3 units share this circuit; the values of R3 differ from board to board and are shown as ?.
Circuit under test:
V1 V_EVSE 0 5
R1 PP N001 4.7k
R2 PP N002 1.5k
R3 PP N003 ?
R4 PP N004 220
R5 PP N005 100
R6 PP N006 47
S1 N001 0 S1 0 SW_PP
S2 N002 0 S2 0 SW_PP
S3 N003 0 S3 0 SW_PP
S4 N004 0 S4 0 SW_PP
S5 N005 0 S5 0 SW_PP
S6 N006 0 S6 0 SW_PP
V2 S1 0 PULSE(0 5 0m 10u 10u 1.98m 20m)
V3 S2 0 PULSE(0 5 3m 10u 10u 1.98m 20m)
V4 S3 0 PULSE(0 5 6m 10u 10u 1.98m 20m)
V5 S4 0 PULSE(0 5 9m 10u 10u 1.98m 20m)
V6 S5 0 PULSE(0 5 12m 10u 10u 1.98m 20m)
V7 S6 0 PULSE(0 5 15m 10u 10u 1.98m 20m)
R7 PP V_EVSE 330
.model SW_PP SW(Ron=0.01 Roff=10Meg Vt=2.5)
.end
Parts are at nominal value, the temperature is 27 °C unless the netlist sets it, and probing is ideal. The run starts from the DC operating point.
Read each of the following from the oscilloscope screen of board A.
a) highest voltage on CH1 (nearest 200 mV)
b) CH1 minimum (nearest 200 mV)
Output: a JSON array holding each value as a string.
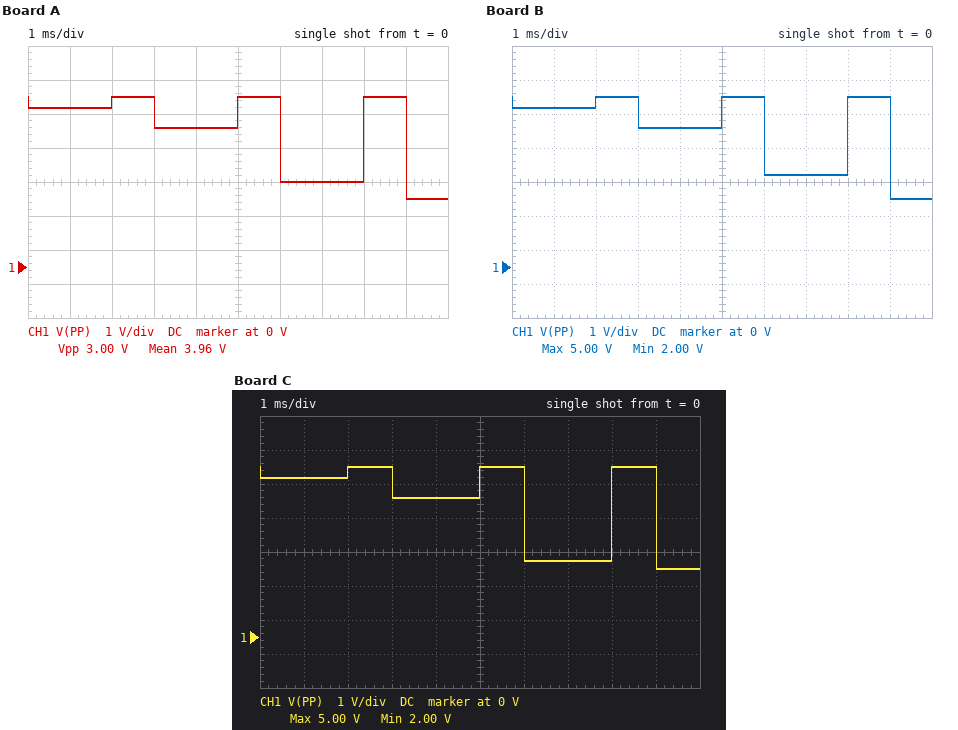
["5.0 V", "2.0 V"]
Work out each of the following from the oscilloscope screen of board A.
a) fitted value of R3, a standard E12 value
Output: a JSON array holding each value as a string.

["330 Ω"]
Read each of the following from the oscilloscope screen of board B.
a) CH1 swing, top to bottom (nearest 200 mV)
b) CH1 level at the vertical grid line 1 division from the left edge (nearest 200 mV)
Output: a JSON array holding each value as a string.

["3.0 V", "4.6 V"]
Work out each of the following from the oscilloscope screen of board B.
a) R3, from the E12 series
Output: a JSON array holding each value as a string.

["390 Ω"]
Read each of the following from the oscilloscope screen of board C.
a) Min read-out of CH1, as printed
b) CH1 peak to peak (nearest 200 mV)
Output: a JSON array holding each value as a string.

["2.00 V", "3.0 V"]
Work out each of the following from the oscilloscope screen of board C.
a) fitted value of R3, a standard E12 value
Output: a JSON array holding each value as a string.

["270 Ω"]
